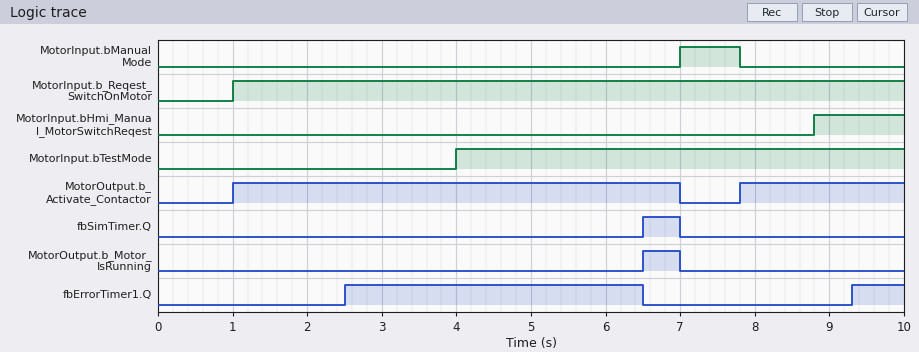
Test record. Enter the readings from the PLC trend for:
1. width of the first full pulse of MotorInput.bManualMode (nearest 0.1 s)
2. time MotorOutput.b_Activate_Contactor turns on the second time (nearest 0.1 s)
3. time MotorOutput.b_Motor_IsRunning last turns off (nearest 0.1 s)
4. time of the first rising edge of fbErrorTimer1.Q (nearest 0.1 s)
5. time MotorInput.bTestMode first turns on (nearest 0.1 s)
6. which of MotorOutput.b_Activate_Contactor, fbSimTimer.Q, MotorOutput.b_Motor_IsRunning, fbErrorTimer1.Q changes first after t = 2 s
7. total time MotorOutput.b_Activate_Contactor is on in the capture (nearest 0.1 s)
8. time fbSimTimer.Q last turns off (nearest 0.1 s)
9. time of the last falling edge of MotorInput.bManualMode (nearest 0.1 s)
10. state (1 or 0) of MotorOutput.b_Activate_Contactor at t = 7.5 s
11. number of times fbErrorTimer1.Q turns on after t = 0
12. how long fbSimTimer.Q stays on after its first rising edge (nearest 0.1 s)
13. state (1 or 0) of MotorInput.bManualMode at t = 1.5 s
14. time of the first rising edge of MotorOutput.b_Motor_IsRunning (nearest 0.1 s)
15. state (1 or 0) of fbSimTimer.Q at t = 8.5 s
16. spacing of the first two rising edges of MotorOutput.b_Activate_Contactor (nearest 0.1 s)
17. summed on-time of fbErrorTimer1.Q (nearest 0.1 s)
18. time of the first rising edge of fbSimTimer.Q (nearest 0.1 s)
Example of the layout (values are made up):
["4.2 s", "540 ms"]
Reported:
["0.8 s", "7.8 s", "7.0 s", "2.5 s", "4.0 s", "fbErrorTimer1.Q", "8.2 s", "7.0 s", "7.8 s", "0", "2", "0.5 s", "0", "6.5 s", "0", "6.8 s", "4.7 s", "6.5 s"]
